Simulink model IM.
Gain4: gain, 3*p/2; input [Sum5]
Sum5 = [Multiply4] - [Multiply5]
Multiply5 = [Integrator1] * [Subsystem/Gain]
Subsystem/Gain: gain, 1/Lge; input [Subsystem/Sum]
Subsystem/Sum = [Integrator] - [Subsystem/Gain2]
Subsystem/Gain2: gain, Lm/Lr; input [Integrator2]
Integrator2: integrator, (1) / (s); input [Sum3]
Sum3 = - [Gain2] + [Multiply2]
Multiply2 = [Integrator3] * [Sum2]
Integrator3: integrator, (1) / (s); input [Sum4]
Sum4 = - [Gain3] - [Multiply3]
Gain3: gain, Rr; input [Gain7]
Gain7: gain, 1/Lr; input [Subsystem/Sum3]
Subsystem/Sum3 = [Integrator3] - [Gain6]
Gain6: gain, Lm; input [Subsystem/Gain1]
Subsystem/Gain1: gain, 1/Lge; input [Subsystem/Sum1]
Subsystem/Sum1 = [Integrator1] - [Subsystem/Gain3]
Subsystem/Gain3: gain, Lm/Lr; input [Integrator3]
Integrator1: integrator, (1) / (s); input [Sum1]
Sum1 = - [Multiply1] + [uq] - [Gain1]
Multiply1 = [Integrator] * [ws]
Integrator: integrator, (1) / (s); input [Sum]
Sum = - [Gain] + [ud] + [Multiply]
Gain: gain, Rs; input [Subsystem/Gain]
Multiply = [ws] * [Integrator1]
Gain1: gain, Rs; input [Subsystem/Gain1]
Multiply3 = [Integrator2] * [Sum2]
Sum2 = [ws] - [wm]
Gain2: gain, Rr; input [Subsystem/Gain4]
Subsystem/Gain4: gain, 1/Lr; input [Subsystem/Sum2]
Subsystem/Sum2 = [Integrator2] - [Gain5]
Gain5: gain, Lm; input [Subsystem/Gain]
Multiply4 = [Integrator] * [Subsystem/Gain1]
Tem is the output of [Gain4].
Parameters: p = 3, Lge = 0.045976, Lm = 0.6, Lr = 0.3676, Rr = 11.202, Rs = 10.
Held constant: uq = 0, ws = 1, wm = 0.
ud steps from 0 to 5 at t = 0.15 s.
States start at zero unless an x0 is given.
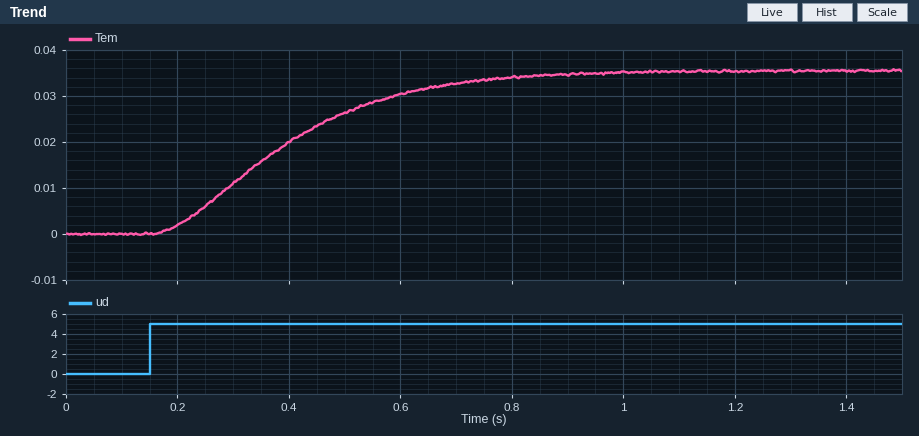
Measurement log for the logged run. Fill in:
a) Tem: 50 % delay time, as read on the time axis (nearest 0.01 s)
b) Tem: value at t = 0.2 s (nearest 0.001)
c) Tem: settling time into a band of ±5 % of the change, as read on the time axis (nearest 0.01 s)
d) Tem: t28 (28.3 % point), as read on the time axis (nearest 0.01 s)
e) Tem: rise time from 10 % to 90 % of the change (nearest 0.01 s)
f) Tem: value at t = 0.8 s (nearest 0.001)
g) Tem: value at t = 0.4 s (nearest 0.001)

0.37 s
0.002
0.77 s
0.29 s
0.44 s
0.034
0.020
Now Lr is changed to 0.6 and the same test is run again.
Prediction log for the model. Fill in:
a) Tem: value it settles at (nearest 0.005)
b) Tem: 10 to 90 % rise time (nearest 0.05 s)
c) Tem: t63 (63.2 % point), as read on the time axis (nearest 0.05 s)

0.035
0.40 s
0.40 s
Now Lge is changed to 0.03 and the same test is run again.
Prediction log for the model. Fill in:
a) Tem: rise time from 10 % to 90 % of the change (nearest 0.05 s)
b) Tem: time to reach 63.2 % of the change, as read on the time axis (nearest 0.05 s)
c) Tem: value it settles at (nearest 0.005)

0.45 s
0.45 s
0.035
